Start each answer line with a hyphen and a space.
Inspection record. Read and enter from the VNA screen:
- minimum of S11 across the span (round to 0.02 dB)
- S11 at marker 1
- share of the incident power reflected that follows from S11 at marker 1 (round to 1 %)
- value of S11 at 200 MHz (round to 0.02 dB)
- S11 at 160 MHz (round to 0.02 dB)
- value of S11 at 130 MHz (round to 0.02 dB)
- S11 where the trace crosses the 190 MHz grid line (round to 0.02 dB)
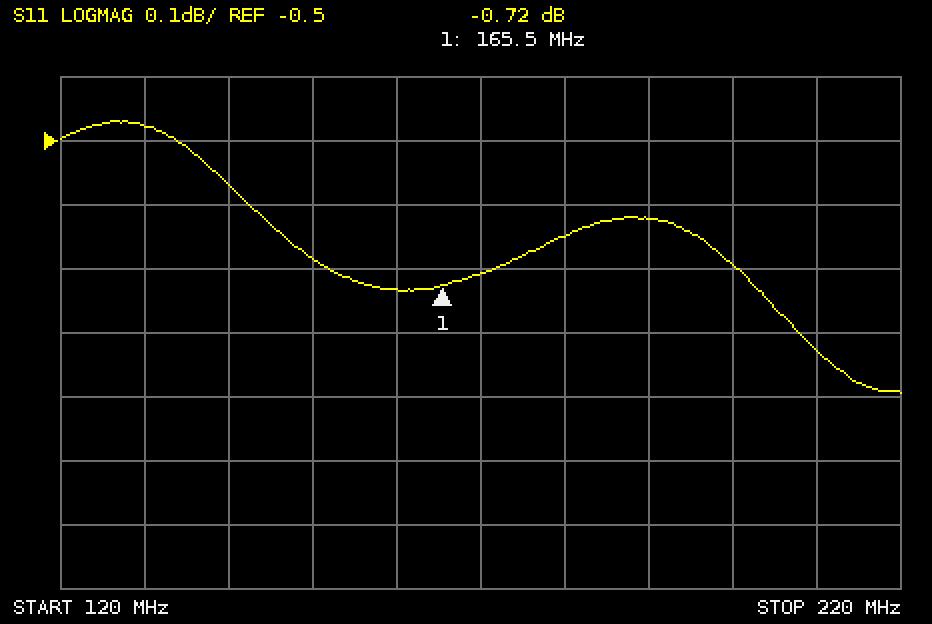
- -0.90 dB
- -0.72 dB
- 85 %
- -0.70 dB
- -0.74 dB
- -0.48 dB
- -0.62 dB
